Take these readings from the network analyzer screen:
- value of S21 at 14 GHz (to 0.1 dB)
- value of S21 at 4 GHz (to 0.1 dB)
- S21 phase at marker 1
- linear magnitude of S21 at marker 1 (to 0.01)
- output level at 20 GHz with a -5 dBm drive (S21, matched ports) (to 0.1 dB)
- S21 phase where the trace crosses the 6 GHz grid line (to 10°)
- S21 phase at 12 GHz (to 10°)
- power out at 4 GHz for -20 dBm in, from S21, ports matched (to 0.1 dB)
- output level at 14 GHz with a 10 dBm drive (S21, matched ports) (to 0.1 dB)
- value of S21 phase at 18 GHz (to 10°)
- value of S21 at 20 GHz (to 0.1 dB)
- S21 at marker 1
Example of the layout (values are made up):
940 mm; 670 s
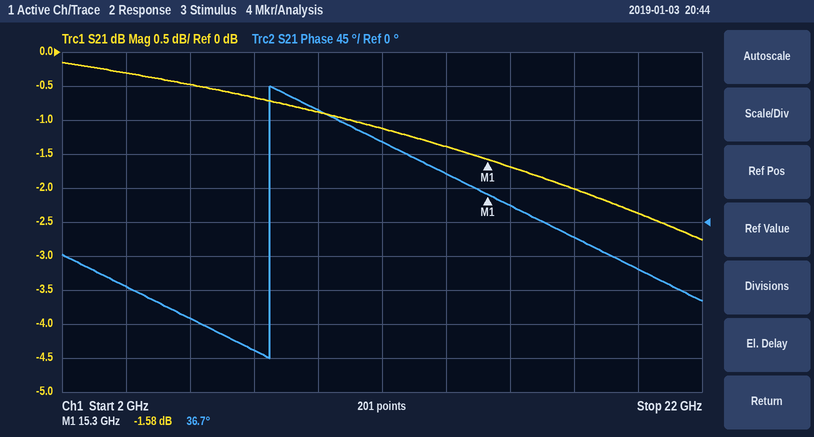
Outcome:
-1.4 dB; -0.3 dB; 36.7°; 0.83; -7.4 dBm; -130°; 110°; -20.3 dBm; 8.6 dBm; -20°; -2.4 dB; -1.58 dB
